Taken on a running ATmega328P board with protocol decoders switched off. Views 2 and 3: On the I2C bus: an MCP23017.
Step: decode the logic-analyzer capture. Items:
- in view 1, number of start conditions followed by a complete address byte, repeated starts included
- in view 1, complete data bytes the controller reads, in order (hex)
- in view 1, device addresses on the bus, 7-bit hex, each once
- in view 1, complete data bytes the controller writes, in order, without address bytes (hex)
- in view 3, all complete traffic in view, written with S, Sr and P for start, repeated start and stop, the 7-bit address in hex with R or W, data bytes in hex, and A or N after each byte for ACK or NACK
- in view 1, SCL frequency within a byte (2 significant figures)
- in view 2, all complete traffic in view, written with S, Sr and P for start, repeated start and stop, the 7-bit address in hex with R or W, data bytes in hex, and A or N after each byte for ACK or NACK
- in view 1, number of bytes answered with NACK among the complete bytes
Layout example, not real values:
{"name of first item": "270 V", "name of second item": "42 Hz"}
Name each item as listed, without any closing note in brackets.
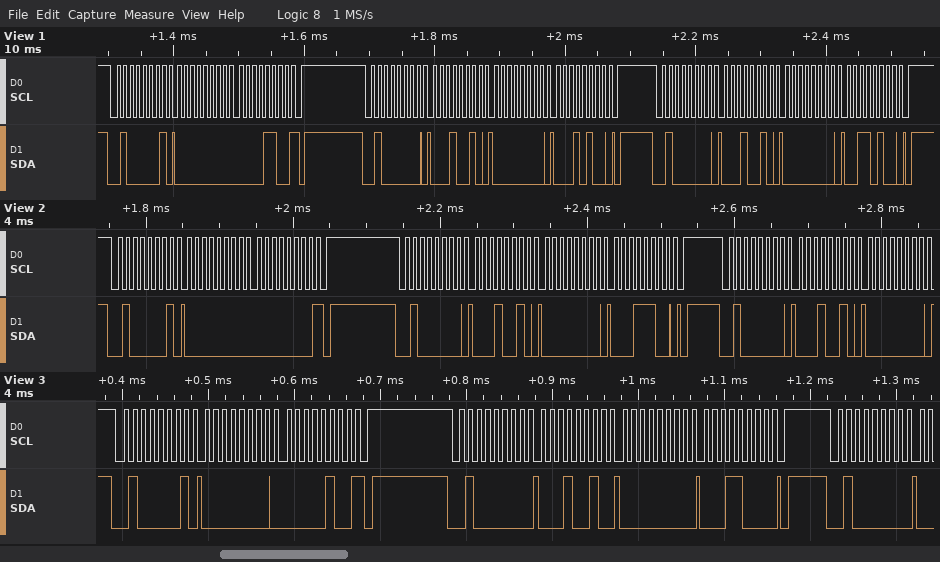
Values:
{"in view 1, number of start conditions followed by a complete address byte, repeated starts included": "3", "in view 1, complete data bytes the controller reads, in order": "00 0C", "in view 1, device addresses on the bus, 7-bit hex, each once": "0x20", "in view 1, complete data bytes the controller writes, in order, without address bytes": "12 00 14 12 00 34", "in view 3, all complete traffic in view, written with S, Sr and P for start, repeated start and stop, the 7-bit address in hex with R or W, data bytes in hex, and A or N after each byte for ACK or NACK": "S 20R A 00 A 04 N P S 20W A 12 A 00 A 18 A P S 20W A", "in view 1, SCL frequency within a byte": "100 kHz", "in view 2, all complete traffic in view, written with S, Sr and P for start, repeated start and stop, the 7-bit address in hex with R or W, data bytes in hex, and A or N after each byte for ACK or NACK": "S 20R A 00 A 00 N P S 20W A 12 A 00 A 1C A P S 20W A 12 A 00 A", "in view 1, number of bytes answered with NACK among the complete bytes": "1"}
